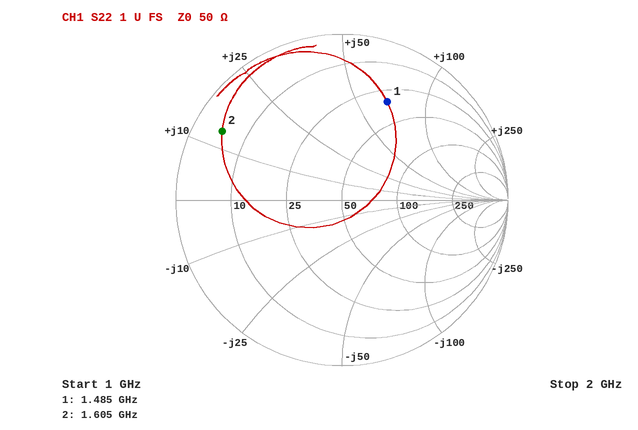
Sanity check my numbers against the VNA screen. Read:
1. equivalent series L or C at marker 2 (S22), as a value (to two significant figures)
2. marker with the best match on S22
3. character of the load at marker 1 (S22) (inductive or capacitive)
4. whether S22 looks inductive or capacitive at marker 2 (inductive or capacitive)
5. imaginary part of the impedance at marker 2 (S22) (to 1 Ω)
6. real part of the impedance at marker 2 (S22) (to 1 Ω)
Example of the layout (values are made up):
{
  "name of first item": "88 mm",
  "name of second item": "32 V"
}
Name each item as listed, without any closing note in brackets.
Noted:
{
  "equivalent series L or C at marker 2 (S22), as a value": "1.3 nH",
  "marker with the best match on S22": "marker 1",
  "character of the load at marker 1 (S22)": "inductive",
  "whether S22 looks inductive or capacitive at marker 2": "inductive",
  "imaginary part of the impedance at marker 2 (S22)": "+13 Ω",
  "real part of the impedance at marker 2 (S22)": "5 Ω"
}
